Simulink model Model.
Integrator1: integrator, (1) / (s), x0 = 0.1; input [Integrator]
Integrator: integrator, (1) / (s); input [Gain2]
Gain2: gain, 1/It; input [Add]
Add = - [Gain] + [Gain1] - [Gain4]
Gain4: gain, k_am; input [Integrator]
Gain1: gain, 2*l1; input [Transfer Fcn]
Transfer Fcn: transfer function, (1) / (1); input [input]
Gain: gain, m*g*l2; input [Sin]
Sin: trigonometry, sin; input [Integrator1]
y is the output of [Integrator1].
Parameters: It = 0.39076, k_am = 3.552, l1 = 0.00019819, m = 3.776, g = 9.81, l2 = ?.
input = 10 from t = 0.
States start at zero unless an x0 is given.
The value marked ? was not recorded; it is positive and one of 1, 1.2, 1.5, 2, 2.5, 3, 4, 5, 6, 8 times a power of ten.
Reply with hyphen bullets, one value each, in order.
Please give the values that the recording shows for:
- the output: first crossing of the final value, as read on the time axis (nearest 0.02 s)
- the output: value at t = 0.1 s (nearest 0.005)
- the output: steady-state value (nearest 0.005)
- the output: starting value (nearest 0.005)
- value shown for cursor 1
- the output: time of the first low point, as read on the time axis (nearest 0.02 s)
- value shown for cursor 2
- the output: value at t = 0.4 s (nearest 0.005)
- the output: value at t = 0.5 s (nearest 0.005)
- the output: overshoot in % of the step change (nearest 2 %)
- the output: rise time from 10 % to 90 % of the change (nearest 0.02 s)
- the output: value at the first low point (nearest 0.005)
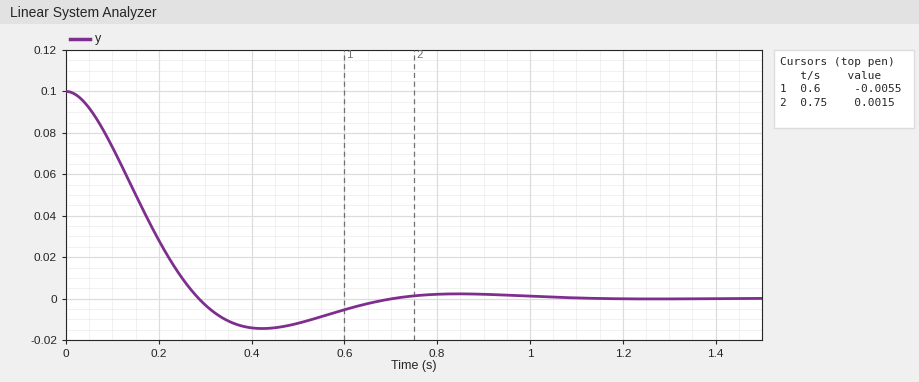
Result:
- 0.28 s
- 0.075
- 0.000
- 0.100
- -0.0055
- 0.42 s
- 0.0015
- -0.015
- -0.010
- 14 %
- 0.20 s
- -0.015
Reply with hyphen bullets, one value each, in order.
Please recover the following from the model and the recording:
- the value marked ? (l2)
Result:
- 0.8
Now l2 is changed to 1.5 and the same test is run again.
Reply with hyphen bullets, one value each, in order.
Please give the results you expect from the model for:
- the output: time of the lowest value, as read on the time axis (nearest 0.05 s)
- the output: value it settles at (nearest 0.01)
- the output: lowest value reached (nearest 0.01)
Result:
- 0.30 s
- 0.00
- -0.03
